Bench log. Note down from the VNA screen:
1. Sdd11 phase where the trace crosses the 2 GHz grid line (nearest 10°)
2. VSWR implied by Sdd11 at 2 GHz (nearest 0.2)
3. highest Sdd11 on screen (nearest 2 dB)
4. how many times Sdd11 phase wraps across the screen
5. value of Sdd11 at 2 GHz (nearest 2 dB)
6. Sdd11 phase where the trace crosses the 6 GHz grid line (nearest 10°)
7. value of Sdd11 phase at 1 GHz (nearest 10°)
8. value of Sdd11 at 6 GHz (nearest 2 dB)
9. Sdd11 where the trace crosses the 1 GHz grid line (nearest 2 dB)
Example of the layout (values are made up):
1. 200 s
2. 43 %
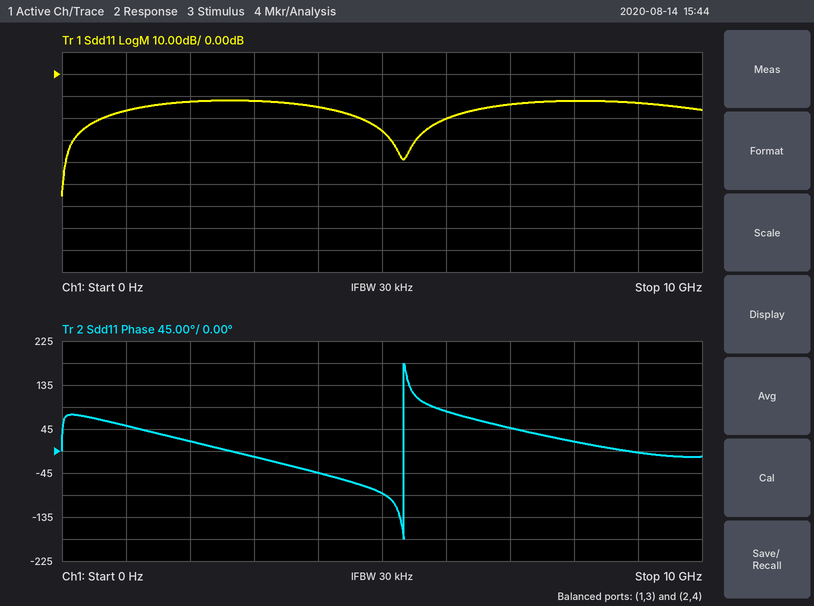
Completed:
1. 20°
2. 1.6
3. -12 dB
4. 1
5. -12 dB
6. 80°
7. 50°
8. -20 dB
9. -16 dB
